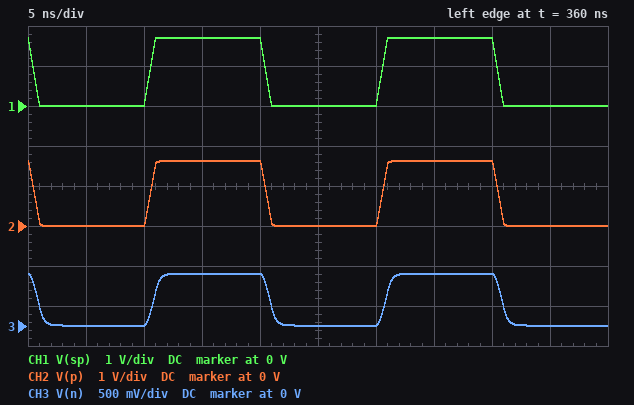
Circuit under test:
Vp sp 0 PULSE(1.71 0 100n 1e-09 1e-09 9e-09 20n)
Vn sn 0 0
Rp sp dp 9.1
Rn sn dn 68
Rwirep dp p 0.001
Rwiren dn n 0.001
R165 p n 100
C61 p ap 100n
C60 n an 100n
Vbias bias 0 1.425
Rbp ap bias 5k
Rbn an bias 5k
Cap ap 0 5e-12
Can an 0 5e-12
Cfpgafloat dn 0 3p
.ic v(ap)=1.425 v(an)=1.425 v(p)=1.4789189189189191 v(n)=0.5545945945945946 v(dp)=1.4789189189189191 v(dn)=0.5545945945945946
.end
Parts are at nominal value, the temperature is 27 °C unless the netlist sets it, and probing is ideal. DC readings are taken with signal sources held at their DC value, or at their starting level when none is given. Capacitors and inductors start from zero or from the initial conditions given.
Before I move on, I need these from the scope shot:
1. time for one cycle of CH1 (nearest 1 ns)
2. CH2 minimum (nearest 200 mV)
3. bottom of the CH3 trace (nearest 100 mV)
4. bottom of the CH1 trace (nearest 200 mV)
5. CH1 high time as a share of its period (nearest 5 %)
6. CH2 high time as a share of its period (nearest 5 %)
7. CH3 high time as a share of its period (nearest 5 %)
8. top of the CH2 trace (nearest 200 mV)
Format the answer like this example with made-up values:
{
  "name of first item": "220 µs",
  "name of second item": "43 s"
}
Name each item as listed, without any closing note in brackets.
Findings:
{
  "time for one cycle of CH1": "20 ns",
  "CH2 minimum": "0 V",
  "bottom of the CH3 trace": "0 V",
  "bottom of the CH1 trace": "0 V",
  "CH1 high time as a share of its period": "50 %",
  "CH2 high time as a share of its period": "50 %",
  "CH3 high time as a share of its period": "50 %",
  "top of the CH2 trace": "1.6 V"
}
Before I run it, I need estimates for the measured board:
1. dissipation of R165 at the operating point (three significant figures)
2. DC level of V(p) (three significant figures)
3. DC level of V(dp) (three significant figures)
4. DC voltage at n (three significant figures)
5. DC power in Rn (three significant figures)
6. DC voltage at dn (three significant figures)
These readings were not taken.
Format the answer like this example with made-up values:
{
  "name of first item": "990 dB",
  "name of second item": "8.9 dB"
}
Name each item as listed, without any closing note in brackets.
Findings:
{
  "dissipation of R165 at the operating point": "9.32 mW",
  "DC level of V(p)": "1.62 V",
  "DC level of V(dp)": "1.62 V",
  "DC voltage at n": "657 mV",
  "DC power in Rn": "6.34 mW",
  "DC voltage at dn": "657 mV"
}
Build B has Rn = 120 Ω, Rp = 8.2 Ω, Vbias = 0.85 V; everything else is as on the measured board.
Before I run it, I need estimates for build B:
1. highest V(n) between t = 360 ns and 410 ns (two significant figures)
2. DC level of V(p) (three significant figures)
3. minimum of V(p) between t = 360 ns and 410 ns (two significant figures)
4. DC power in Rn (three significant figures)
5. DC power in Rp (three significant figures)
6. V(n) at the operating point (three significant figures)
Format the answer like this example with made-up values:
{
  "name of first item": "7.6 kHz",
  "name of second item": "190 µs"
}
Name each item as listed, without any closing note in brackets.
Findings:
{
  "highest V(n) between t = 360 ns and 410 ns": "890 mV",
  "DC level of V(p)": "1.65 V",
  "minimum of V(p) between t = 360 ns and 410 ns": "1.4 mV",
  "DC power in Rn": "6.74 mW",
  "DC power in Rp": "460 µW",
  "V(n) at the operating point": "899 mV"
}
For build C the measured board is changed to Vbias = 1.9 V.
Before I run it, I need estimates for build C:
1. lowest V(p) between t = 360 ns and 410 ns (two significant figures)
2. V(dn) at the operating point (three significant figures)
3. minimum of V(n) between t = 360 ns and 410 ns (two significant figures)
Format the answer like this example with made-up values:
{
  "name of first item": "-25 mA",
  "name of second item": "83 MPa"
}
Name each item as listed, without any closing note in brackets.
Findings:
{
  "lowest V(p) between t = 360 ns and 410 ns": "4.1 mV",
  "V(dn) at the operating point": "657 mV",
  "minimum of V(n) between t = 360 ns and 410 ns": "9.9 mV"
}
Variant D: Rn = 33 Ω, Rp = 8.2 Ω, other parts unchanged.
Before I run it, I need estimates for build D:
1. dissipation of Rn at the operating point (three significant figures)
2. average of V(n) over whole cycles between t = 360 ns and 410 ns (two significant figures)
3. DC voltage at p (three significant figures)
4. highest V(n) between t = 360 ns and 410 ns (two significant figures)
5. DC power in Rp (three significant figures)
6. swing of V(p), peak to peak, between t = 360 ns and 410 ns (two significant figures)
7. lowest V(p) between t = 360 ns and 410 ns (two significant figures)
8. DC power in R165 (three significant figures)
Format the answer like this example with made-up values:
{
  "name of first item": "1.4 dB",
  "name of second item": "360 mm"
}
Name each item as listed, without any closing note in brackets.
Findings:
{
  "dissipation of Rn at the operating point": "4.84 mW",
  "average of V(n) over whole cycles between t = 360 ns and 410 ns": "200 mV",
  "DC voltage at p": "1.61 V",
  "highest V(n) between t = 360 ns and 410 ns": "400 mV",
  "DC power in Rp": "1.20 mW",
  "swing of V(p), peak to peak, between t = 360 ns and 410 ns": "1.6 V",
  "lowest V(p) between t = 360 ns and 410 ns": "2.5 mV",
  "DC power in R165": "14.7 mW"
}
